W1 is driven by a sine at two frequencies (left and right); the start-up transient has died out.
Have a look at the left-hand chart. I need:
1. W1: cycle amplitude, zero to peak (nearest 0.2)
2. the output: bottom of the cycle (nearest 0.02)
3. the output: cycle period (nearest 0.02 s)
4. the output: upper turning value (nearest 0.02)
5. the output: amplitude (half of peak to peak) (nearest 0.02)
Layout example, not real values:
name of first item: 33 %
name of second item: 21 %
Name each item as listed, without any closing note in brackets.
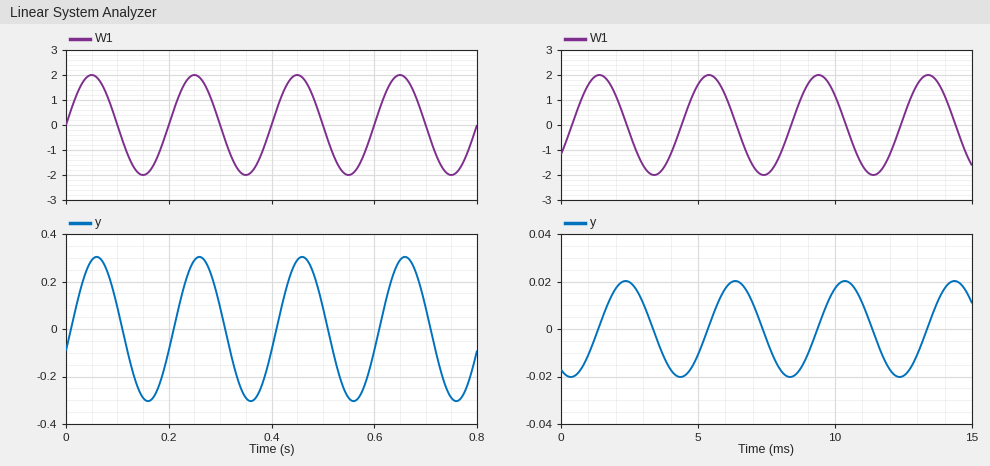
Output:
W1: cycle amplitude, zero to peak: 2.0
the output: bottom of the cycle: -0.30
the output: cycle period: 0.20 s
the output: upper turning value: 0.30
the output: amplitude (half of peak to peak): 0.30
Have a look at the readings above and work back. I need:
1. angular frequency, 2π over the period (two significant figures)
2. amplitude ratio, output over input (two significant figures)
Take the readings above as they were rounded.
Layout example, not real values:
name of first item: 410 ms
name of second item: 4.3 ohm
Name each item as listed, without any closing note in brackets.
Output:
angular frequency, 2π over the period: 31 rad/s
amplitude ratio, output over input: 0.15
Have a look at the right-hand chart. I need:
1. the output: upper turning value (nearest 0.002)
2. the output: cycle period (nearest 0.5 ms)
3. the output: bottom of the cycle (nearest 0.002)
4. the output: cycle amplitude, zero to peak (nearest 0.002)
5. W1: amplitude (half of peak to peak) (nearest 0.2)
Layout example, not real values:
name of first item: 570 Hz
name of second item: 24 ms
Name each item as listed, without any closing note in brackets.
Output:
the output: upper turning value: 0.020
the output: cycle period: 4.0 ms
the output: bottom of the cycle: -0.020
the output: cycle amplitude, zero to peak: 0.020
W1: amplitude (half of peak to peak): 2.0
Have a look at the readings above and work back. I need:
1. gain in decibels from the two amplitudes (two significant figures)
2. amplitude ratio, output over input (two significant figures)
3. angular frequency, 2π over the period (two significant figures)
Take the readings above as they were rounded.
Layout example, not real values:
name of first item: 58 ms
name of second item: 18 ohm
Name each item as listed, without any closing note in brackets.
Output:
gain in decibels from the two amplitudes: -40 dB
amplitude ratio, output over input: 0.010
angular frequency, 2π over the period: 1.6 rad/ms
